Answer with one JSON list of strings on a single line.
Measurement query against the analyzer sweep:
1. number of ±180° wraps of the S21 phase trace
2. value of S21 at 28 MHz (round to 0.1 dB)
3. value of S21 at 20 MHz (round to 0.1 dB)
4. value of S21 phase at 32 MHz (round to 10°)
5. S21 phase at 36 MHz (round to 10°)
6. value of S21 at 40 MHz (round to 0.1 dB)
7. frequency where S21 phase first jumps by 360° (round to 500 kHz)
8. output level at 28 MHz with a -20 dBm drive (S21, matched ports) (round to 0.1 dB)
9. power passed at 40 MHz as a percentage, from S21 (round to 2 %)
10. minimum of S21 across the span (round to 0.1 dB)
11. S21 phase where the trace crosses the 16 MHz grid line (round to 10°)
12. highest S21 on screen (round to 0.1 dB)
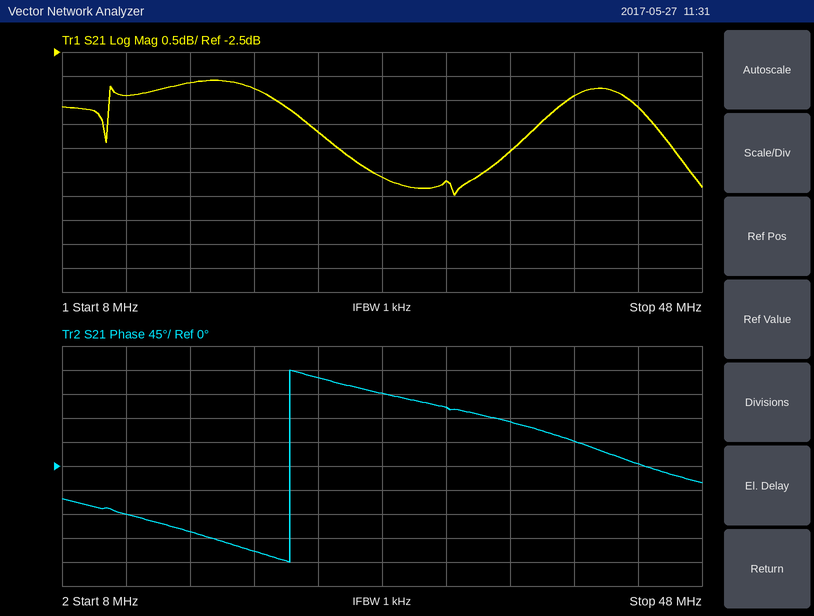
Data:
["1", "-5.1 dB", "-3.3 dB", "110°", "80°", "-3.4 dB", "22.0 MHz", "-25.1 dBm", "46 %", "-5.5 dB", "-120°", "-3.1 dB"]
